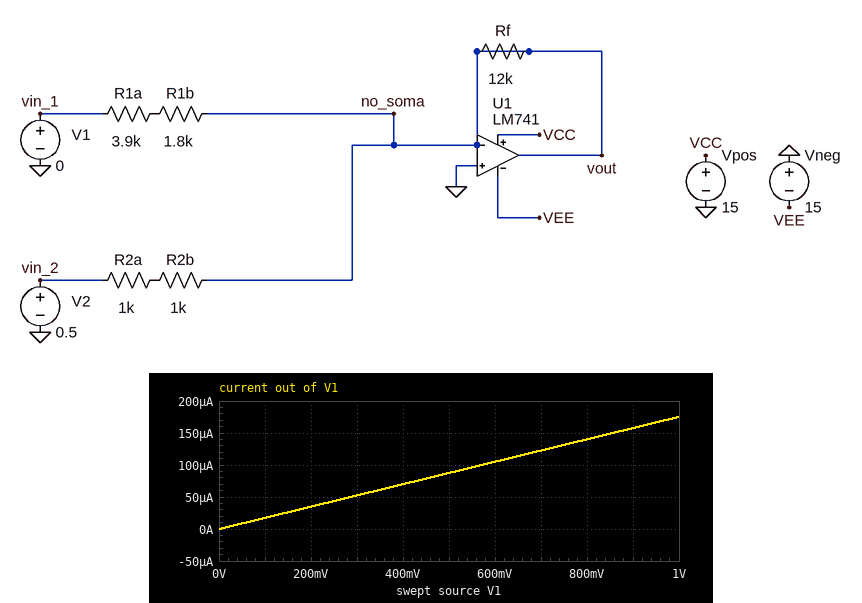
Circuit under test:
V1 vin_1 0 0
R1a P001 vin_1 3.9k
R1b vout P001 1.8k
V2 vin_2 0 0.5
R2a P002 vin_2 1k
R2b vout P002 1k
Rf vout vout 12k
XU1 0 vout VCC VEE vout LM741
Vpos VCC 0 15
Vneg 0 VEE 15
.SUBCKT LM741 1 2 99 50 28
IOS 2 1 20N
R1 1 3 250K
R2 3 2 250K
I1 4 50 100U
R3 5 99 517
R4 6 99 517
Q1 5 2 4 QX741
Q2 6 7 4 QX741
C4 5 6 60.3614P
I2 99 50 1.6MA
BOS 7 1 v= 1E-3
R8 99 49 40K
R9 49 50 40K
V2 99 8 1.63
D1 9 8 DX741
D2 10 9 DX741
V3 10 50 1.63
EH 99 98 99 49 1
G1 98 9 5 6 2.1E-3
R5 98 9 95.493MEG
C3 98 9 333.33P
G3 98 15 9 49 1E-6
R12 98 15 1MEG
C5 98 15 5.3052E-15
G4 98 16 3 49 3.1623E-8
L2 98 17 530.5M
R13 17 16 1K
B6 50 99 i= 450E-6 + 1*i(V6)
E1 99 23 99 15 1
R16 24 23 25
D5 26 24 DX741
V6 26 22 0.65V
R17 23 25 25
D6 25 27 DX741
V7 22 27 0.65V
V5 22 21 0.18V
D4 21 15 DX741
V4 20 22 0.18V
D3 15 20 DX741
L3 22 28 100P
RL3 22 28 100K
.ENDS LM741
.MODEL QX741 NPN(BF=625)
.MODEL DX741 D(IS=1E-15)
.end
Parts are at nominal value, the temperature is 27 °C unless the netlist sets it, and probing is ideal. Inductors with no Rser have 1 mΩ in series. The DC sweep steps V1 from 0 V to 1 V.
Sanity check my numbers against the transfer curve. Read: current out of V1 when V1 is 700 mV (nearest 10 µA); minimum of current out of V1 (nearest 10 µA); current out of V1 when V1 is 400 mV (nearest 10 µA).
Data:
120 µA
0 A
70 µA
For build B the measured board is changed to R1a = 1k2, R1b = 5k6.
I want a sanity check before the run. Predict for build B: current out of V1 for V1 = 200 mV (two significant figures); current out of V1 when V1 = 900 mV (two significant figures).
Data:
29 µA
130 µA
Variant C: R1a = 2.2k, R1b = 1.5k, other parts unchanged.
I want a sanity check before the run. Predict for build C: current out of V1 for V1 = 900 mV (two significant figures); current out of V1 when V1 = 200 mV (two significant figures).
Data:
240 µA
54 µA
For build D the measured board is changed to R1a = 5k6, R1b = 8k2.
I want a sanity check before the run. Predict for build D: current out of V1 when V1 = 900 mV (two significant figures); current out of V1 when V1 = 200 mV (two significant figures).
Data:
65 µA
14 µA
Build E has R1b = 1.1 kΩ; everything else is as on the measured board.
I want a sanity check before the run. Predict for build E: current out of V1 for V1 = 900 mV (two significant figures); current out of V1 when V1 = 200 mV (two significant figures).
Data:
180 µA
40 µA
